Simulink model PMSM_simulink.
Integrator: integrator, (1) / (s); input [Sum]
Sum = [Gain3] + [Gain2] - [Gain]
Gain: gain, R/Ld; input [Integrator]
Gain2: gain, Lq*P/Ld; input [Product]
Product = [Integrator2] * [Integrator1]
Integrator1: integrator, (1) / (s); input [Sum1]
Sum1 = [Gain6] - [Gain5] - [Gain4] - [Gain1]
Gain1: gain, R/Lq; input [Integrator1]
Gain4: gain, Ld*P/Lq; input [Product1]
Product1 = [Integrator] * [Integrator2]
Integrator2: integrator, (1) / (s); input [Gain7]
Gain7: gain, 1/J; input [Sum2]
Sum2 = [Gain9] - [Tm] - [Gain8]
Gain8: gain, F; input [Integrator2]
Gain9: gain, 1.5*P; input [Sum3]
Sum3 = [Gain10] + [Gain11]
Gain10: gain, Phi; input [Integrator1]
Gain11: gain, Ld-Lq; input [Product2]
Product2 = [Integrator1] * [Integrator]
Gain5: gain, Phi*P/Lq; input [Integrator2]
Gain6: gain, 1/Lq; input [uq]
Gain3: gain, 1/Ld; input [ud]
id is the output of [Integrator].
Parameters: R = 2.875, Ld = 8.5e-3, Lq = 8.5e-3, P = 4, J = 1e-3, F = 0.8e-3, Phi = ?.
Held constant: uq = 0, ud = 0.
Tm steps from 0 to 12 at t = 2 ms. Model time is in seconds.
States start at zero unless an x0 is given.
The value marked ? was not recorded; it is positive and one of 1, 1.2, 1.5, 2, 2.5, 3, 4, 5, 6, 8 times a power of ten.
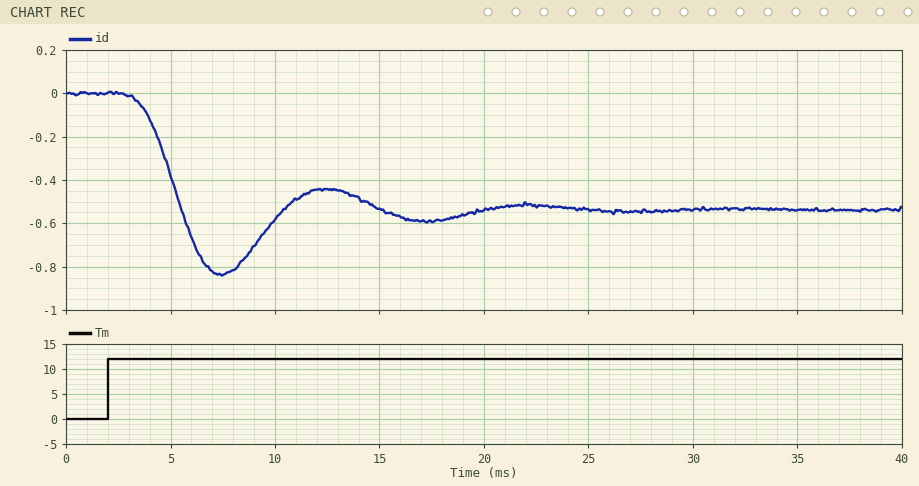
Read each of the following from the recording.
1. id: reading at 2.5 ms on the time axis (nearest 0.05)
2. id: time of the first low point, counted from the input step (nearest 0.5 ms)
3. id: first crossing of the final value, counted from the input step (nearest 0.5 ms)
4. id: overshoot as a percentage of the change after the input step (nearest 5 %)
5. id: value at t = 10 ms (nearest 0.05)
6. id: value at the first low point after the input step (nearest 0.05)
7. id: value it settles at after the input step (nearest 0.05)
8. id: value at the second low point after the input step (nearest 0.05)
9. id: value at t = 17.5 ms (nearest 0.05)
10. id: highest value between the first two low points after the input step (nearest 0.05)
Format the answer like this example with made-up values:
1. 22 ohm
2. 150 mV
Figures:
1. 0.00
2. 5.5 ms
3. 3.5 ms
4. 55 %
5. -0.60
6. -0.85
7. -0.55
8. -0.60
9. -0.60
10. -0.45
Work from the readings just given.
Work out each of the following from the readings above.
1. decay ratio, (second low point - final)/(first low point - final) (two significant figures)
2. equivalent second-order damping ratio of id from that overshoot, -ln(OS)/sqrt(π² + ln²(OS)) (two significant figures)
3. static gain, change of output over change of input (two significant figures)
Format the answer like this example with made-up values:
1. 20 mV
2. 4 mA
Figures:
1. 0.17
2. 0.19
3. -0.046
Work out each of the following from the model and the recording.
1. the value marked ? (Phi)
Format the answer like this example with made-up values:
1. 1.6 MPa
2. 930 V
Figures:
1. 0.4
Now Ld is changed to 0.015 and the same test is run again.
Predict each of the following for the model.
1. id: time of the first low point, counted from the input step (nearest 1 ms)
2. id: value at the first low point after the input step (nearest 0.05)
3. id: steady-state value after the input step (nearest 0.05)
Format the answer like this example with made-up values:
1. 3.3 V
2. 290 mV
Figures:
1. 6 ms
2. -0.60
3. -0.55
